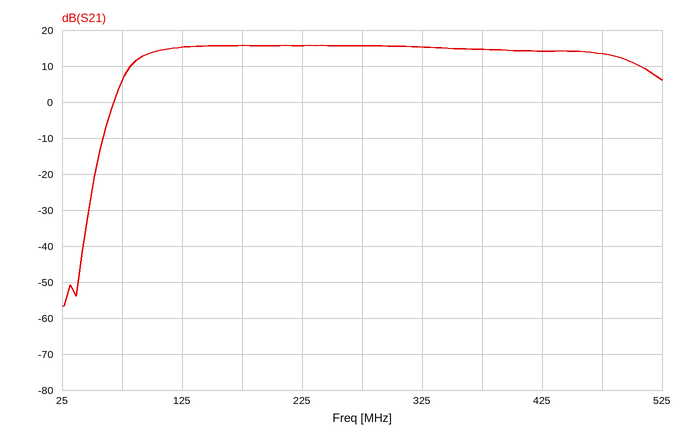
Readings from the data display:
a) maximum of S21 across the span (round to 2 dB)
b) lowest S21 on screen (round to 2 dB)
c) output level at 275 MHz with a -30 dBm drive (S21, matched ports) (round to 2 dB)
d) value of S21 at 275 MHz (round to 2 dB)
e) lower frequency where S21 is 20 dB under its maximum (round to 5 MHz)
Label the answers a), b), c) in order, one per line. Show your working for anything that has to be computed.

a) 16 dB
b) -56 dB
c) -30 dBm + (16 dB) = -14 dBm
d) 16 dB
e) 65 MHz
